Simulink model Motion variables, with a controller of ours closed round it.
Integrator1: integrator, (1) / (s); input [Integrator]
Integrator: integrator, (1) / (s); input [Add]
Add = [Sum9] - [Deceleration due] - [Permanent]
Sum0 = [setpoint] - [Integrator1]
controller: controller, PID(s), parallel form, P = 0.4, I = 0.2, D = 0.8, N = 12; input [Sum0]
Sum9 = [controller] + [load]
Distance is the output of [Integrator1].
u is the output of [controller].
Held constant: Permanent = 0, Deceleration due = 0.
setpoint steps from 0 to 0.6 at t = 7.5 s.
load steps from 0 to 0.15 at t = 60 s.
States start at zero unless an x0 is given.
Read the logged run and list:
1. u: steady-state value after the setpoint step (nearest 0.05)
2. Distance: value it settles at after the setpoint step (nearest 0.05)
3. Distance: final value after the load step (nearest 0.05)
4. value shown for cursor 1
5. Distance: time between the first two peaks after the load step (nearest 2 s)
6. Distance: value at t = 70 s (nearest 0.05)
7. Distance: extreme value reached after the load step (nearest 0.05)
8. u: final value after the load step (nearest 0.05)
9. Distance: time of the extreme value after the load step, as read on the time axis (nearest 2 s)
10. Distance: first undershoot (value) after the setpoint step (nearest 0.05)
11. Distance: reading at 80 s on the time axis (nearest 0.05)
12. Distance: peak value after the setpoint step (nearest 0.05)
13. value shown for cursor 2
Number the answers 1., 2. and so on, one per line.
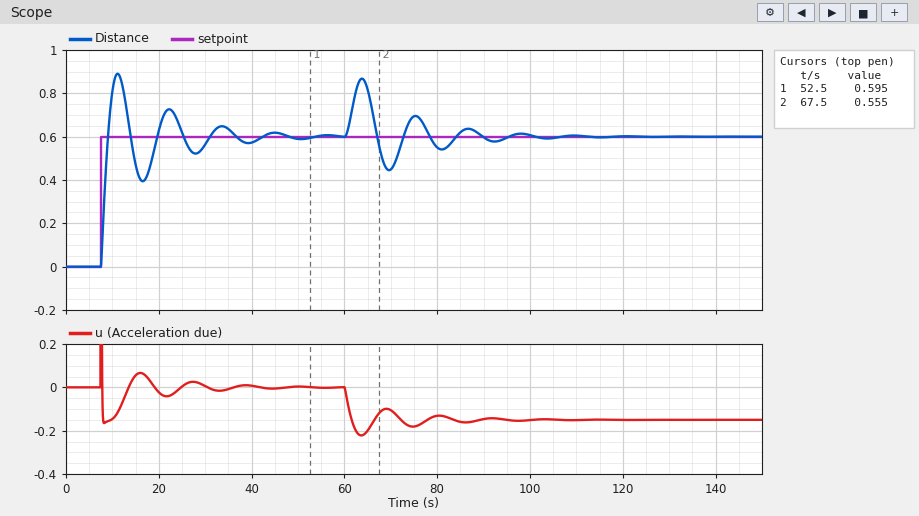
1. 0.00
2. 0.60
3. 0.60
4. 0.595
5. 12 s
6. 0.45
7. 0.85
8. -0.15
9. 64 s
10. 0.40
11. 0.55
12. 0.90
13. 0.555
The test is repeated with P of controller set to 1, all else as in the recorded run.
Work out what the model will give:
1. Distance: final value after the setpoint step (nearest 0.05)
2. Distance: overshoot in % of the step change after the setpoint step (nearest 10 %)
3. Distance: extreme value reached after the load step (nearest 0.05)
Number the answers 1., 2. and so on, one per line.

1. 0.60
2. 50 %
3. 0.75
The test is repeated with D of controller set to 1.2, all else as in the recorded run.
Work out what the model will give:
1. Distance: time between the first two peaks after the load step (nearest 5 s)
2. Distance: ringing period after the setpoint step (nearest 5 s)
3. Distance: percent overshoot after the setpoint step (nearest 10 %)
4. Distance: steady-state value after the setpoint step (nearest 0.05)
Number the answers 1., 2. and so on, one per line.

1. 15 s
2. 15 s
3. 30 %
4. 0.60
